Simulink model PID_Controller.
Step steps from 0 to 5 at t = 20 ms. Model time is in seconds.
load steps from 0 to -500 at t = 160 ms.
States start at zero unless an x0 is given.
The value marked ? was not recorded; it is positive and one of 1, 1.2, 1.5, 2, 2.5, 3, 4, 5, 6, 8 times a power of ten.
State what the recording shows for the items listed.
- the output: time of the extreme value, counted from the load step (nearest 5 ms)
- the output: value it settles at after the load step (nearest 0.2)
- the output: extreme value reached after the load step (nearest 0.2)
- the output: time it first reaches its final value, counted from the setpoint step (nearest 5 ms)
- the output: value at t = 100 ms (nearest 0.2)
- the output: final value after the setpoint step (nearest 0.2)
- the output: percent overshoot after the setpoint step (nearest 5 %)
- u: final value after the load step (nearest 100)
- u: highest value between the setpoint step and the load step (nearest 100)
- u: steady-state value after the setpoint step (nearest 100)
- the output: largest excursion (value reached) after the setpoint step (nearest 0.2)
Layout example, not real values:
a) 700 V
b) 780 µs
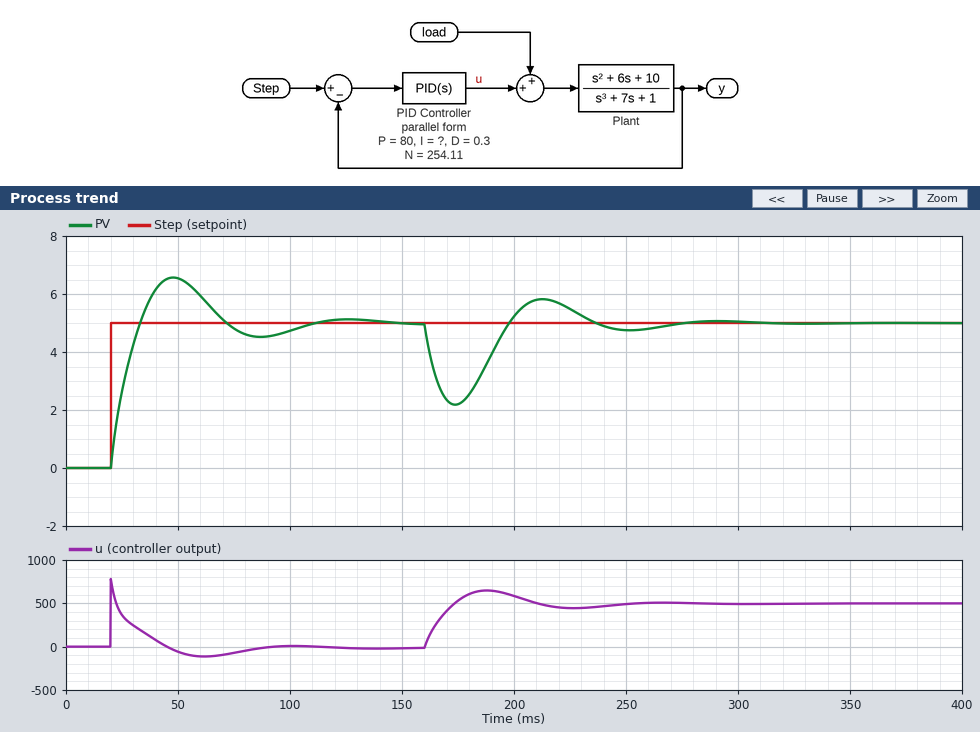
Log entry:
a) 15 ms
b) 5.0
c) 2.2
d) 15 ms
e) 4.8
f) 5.0
g) 30 %
h) 500
i) 800
j) 0
k) 6.6
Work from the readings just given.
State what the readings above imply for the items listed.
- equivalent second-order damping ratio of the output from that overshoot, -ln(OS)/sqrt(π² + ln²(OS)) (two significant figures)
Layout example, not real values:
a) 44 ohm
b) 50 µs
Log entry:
a) 0.36
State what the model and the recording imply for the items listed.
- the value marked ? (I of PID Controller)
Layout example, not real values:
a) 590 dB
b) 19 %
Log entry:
a) 10000
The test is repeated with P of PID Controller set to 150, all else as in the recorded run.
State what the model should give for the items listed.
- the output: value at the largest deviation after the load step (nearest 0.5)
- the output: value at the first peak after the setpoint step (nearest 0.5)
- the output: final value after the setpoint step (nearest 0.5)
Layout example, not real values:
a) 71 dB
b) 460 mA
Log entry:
a) 3.0
b) 6.0
c) 5.0
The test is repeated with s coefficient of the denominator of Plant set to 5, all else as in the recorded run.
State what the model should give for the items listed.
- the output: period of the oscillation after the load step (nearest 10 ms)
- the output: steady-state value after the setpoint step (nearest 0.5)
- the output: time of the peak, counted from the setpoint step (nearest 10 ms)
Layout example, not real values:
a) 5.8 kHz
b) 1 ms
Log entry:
a) 80 ms
b) 5.0
c) 30 ms
